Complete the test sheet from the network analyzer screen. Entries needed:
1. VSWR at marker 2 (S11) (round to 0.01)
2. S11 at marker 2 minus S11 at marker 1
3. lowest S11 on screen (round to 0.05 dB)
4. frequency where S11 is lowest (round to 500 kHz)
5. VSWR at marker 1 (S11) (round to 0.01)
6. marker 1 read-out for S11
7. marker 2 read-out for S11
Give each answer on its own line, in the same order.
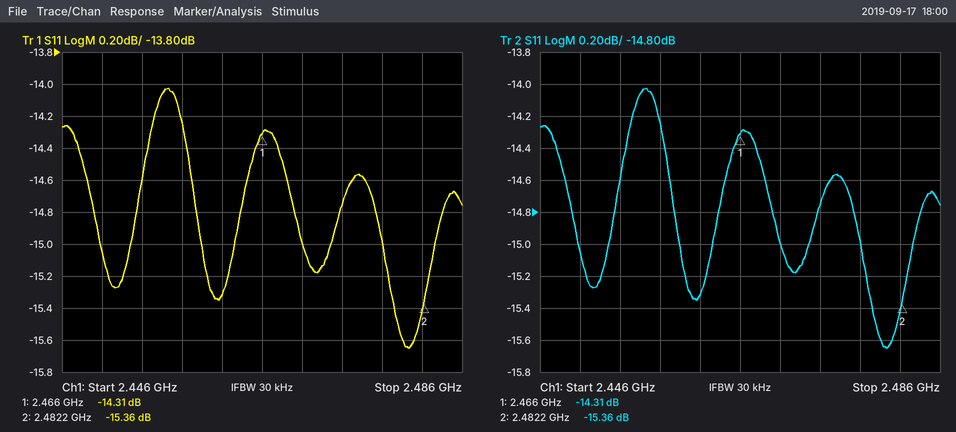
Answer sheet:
1.41
-1.05 dB
-15.65 dB
2.4805 GHz
1.48
-14.31 dB
-15.36 dB
